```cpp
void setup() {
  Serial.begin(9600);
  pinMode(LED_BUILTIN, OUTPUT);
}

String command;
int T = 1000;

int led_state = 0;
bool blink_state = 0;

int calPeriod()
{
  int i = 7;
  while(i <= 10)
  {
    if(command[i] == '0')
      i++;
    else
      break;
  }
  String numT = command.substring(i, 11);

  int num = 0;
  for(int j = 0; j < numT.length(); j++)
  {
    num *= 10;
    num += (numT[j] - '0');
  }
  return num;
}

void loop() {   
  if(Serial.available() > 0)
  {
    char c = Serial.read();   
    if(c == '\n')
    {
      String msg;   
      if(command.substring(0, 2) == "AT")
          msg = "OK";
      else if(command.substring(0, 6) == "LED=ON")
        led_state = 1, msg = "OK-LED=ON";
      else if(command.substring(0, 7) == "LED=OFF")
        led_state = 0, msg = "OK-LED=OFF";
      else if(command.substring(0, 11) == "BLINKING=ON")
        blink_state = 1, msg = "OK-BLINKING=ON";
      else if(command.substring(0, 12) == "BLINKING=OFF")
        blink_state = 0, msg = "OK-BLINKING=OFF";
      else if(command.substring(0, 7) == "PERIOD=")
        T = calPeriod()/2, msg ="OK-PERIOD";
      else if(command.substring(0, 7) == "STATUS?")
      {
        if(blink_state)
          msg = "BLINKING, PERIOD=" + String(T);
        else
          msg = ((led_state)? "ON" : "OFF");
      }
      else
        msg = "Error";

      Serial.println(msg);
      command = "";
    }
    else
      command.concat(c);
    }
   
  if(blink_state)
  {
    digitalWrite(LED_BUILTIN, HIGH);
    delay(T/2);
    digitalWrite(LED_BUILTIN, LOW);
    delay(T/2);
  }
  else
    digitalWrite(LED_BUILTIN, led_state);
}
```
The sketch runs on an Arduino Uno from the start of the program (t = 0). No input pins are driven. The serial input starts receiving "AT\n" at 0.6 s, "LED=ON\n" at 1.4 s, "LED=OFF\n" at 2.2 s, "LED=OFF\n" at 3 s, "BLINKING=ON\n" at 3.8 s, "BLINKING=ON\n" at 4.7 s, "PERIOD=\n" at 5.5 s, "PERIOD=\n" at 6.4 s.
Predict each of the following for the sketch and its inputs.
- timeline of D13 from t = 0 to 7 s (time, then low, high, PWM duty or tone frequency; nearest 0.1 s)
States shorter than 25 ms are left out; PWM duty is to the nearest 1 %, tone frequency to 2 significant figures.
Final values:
0 s low; 1.4 s high; 2.2 s low; 3.8 s high; 4.3 s low; 4.8 s high; 5.3 s low; 5.8 s high; 6.3 s low; 6.8 s high
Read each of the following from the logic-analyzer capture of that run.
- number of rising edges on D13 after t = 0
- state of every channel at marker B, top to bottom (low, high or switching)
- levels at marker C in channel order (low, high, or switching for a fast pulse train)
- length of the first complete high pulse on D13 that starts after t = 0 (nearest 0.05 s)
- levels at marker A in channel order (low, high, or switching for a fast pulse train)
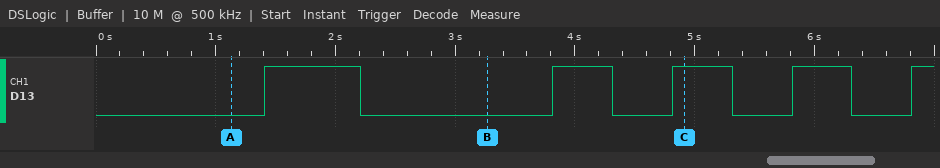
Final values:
5
D13 low
D13 high
0.80 s
D13 low
